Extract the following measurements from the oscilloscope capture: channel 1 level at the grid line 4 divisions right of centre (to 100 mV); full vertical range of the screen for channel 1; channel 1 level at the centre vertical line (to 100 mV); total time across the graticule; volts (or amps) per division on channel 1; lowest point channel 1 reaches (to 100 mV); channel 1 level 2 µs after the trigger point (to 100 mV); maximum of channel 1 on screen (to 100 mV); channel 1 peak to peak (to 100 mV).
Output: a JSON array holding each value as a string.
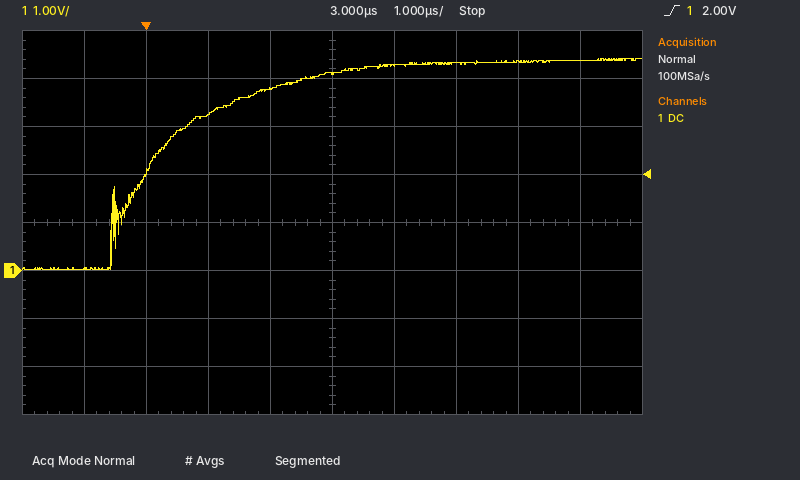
["4.4 V", "8 V", "4.1 V", "10 µs", "1 V", "0.0 V", "3.8 V", "4.4 V", "4.4 V"]
